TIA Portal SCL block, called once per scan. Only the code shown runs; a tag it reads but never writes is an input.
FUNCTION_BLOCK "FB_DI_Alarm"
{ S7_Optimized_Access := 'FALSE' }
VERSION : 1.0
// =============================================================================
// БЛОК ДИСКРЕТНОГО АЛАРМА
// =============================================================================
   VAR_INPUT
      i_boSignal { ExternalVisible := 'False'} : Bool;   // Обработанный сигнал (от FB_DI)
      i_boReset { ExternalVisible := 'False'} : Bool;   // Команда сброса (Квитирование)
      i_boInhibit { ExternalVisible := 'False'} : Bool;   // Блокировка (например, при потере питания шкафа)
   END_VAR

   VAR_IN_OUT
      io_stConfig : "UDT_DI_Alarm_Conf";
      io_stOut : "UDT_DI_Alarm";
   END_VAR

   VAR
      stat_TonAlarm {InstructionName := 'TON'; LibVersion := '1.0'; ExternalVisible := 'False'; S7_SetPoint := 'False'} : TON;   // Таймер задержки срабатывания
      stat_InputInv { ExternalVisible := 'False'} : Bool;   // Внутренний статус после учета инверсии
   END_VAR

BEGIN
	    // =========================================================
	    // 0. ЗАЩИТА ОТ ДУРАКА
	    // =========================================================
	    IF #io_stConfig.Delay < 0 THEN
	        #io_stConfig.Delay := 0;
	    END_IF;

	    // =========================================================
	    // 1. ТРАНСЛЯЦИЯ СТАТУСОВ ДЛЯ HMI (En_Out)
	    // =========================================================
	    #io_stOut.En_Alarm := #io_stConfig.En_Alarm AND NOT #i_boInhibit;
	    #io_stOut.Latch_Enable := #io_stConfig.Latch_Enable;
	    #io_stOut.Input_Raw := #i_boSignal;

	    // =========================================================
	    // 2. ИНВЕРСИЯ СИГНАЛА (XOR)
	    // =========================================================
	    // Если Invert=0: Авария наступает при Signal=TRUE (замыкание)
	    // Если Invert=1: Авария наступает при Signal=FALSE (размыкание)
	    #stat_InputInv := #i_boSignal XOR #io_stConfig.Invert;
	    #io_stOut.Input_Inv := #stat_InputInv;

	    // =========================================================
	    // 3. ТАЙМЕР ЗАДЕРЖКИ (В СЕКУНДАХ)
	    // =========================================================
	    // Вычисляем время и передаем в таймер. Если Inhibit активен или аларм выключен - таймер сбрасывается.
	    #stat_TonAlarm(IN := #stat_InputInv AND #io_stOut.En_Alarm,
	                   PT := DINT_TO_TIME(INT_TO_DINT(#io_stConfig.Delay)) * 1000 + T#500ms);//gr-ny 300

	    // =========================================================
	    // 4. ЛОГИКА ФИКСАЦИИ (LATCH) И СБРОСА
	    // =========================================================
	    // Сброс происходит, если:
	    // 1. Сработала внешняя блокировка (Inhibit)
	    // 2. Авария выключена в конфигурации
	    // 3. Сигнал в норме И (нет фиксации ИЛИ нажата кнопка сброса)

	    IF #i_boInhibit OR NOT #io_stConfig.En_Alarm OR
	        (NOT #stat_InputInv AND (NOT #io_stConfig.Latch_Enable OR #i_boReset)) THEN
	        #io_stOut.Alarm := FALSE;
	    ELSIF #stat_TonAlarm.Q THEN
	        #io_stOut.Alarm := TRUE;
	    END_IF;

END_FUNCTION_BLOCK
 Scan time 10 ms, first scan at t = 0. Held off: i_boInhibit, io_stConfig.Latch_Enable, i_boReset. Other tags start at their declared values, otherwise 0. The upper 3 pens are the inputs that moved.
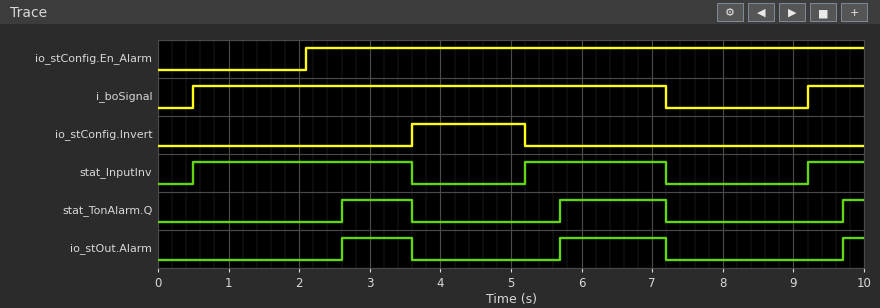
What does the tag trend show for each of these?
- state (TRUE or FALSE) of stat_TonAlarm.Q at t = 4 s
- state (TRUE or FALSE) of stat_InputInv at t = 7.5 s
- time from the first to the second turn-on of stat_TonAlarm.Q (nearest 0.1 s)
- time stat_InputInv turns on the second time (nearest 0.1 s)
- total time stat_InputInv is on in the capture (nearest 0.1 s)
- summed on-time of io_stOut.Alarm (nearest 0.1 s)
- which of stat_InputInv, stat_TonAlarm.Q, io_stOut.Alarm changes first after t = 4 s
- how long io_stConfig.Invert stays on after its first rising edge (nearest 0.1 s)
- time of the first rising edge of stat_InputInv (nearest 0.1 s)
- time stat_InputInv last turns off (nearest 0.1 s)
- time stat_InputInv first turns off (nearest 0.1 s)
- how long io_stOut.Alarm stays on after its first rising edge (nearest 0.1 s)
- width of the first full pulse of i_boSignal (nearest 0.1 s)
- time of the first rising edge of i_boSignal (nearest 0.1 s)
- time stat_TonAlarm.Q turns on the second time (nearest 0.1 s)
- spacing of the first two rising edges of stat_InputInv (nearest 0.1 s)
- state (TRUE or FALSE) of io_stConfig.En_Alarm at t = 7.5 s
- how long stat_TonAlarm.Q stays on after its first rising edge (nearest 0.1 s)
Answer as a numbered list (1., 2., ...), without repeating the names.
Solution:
1. FALSE
2. FALSE
3. 3.1 s
4. 5.2 s
5. 5.9 s
6. 2.8 s
7. stat_InputInv
8. 1.6 s
9. 0.5 s
10. 7.2 s
11. 3.6 s
12. 1.0 s
13. 6.7 s
14. 0.5 s
15. 5.7 s
16. 4.7 s
17. TRUE
18. 1.0 s
